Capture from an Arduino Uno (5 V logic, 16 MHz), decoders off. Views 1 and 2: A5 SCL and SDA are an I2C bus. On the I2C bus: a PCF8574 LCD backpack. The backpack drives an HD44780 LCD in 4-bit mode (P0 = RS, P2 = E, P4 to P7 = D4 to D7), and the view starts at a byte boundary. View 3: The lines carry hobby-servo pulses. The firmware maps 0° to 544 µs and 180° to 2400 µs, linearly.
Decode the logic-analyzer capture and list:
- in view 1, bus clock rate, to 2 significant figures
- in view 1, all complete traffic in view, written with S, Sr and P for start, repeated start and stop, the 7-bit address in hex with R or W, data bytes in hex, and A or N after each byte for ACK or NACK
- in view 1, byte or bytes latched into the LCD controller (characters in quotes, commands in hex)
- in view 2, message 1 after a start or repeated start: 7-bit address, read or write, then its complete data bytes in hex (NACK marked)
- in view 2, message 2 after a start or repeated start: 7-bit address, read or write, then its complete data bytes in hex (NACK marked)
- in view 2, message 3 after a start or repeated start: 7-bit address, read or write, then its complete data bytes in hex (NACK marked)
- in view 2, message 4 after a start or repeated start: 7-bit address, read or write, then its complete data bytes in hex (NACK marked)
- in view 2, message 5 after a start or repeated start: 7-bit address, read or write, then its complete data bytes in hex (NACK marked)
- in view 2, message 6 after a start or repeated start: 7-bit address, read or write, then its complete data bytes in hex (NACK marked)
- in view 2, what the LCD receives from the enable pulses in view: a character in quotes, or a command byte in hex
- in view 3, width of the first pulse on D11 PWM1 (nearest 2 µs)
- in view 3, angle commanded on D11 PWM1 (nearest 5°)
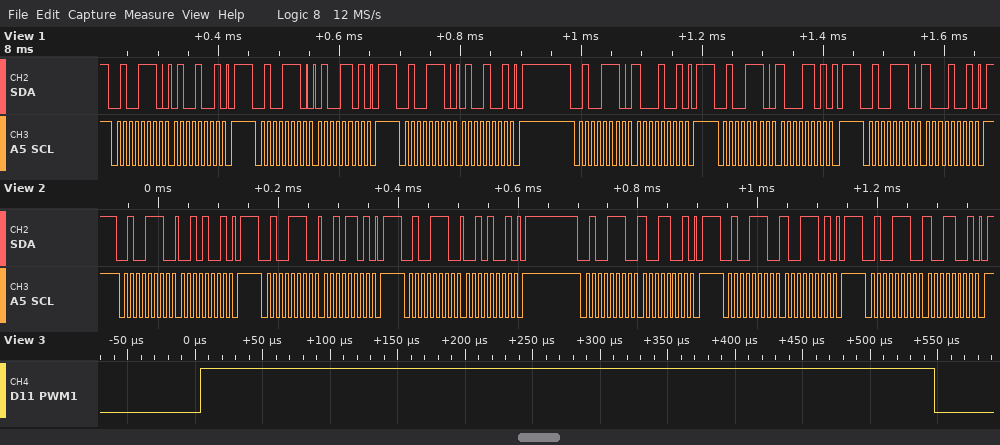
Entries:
100 kHz
S 27W A 49 A P S 27W A 4D A P S 27W A 49 A P S 27W A 89 A P S 27W A 8D A P S 27W A 89 A P
'H'
0x27 write: 29
0x27 write: 2D
0x27 write: 29
0x27 write: 99
0x27 write: 9D
0x27 write: 99
')'
544 µs
0°
